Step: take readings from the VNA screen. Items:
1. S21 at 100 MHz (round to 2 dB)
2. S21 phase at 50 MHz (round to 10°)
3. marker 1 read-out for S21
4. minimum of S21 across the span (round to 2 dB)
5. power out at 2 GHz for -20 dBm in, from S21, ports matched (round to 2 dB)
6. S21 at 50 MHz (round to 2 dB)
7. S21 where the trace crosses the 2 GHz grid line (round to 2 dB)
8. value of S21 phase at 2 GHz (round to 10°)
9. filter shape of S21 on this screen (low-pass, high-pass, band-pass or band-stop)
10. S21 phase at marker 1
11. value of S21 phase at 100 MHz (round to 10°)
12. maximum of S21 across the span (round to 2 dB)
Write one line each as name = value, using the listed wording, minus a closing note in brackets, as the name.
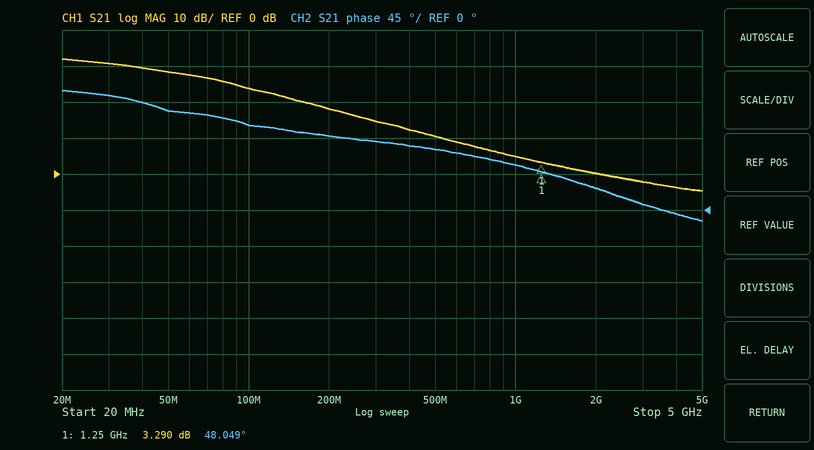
S21 at 100 MHz = 24 dB
S21 phase at 50 MHz = 120°
marker 1 read-out for S21 = 3.290 dB
minimum of S21 across the span = -4 dB
power out at 2 GHz for -20 dBm in, from S21, ports matched = -20 dBm
S21 at 50 MHz = 28 dB
S21 where the trace crosses the 2 GHz grid line = 0 dB
value of S21 phase at 2 GHz = 30°
filter shape of S21 on this screen = low-pass
S21 phase at marker 1 = 48.049°
value of S21 phase at 100 MHz = 110°
maximum of S21 across the span = 32 dB
